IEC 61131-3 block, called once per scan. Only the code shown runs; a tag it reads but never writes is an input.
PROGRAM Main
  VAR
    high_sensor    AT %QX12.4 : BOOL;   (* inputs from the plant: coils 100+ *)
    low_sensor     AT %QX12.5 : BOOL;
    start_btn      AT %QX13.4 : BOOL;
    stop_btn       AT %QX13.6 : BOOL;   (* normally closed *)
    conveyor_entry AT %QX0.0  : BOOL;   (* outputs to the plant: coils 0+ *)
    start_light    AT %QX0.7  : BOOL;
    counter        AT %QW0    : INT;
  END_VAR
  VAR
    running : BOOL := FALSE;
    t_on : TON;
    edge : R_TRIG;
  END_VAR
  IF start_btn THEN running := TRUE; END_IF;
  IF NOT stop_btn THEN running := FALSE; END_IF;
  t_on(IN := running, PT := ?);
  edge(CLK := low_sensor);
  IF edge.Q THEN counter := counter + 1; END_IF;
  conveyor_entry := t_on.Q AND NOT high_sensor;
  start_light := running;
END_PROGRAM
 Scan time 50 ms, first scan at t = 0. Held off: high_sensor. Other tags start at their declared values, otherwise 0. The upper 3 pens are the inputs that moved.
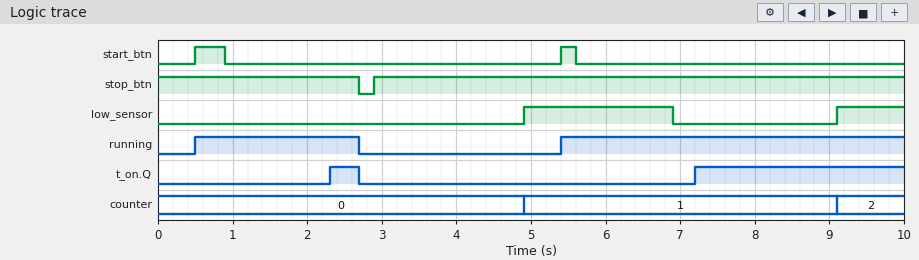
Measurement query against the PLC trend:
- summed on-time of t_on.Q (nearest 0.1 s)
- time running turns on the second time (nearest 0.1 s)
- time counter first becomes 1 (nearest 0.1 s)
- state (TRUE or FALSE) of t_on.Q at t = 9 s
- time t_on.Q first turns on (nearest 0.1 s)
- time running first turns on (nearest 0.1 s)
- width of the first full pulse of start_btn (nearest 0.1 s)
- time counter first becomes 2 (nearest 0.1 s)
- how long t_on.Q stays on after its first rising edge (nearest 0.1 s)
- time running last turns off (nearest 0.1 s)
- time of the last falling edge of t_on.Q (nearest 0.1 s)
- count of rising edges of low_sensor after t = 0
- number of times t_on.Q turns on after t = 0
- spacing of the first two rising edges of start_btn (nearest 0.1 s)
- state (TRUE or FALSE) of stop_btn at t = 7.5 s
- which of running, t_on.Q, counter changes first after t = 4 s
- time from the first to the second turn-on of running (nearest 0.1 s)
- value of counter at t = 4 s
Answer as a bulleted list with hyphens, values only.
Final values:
- 3.2 s
- 5.4 s
- 4.9 s
- TRUE
- 2.3 s
- 0.5 s
- 0.4 s
- 9.1 s
- 0.4 s
- 2.7 s
- 2.7 s
- 2
- 2
- 4.9 s
- TRUE
- counter
- 4.9 s
- 0
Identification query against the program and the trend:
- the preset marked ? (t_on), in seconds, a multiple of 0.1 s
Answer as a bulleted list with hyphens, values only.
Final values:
- 1.8 s
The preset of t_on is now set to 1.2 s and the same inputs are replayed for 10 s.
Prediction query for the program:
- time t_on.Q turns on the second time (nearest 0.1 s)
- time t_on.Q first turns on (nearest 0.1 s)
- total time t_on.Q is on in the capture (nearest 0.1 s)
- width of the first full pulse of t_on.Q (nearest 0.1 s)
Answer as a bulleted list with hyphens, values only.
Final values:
- 6.6 s
- 1.7 s
- 4.4 s
- 1.0 s
